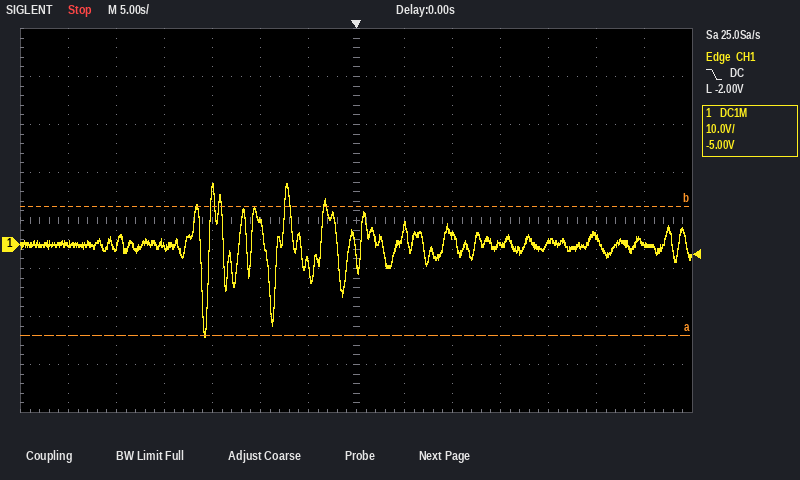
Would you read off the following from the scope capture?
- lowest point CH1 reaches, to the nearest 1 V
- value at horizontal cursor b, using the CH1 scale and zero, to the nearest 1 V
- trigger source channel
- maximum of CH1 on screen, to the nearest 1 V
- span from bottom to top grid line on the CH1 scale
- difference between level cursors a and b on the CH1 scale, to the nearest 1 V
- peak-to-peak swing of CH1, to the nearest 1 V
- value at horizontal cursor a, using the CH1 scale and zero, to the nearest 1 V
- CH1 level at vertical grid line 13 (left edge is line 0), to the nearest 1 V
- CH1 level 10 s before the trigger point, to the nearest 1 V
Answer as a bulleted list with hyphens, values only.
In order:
- -19 V
- 8 V
- CH1
- 13 V
- 80 V
- 27 V
- 32 V
- -19 V
- 0 V
- 5 V
